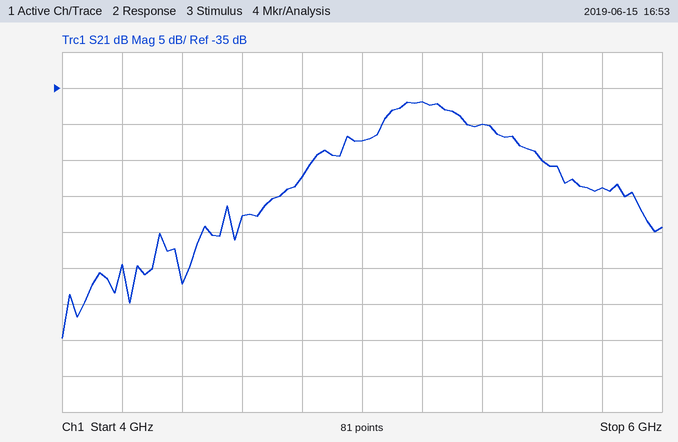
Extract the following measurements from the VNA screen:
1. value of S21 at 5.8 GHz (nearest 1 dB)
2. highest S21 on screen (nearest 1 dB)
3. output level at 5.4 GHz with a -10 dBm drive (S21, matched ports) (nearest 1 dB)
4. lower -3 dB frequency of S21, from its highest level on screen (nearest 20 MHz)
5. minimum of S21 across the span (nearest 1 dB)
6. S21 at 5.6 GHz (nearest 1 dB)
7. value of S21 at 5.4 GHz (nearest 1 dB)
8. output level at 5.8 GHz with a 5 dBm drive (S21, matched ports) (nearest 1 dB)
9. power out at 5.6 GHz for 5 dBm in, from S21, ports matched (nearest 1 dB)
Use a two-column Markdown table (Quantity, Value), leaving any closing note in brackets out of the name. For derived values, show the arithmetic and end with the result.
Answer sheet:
| Quantity | Value |
|---|---|
| value of S21 at 5.8 GHz | -49 dB |
| highest S21 on screen | -37 dB |
| output level at 5.4 GHz with a -10 dBm drive (S21, matched ports) | -10 dBm + (-40 dB) = -50 dBm |
| lower -3 dB frequency of S21, from its highest level on screen | 5.06 GHz |
| minimum of S21 across the span | -70 dB |
| S21 at 5.6 GHz | -45 dB |
| value of S21 at 5.4 GHz | -40 dB |
| output level at 5.8 GHz with a 5 dBm drive (S21, matched ports) | 5 dBm + (-49 dB) = -44 dBm |
| power out at 5.6 GHz for 5 dBm in, from S21, ports matched | 5 dBm + (-45 dB) = -40 dBm |
